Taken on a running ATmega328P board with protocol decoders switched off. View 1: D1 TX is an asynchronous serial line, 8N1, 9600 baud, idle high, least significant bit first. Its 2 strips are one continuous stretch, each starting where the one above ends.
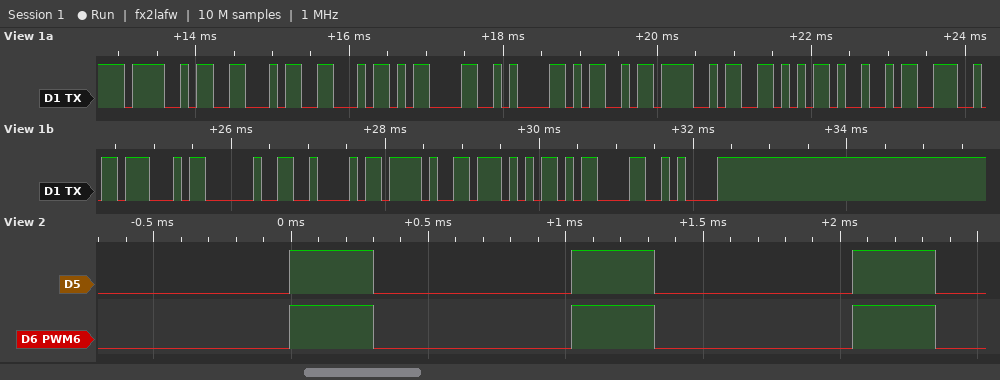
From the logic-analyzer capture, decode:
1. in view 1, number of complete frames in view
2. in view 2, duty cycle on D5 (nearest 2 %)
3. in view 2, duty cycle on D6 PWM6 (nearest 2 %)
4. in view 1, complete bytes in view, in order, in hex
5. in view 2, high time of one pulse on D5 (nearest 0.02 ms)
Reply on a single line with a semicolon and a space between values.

17; 30 %; 30 %; 0x4F 0x46 0x46 0x0D 0x0A 0x4D 0x4F 0x56 0x49 0x4E 0x47 0x20 0x42 0x2F 0x57 0x0D 0x0A; 0.30 ms
